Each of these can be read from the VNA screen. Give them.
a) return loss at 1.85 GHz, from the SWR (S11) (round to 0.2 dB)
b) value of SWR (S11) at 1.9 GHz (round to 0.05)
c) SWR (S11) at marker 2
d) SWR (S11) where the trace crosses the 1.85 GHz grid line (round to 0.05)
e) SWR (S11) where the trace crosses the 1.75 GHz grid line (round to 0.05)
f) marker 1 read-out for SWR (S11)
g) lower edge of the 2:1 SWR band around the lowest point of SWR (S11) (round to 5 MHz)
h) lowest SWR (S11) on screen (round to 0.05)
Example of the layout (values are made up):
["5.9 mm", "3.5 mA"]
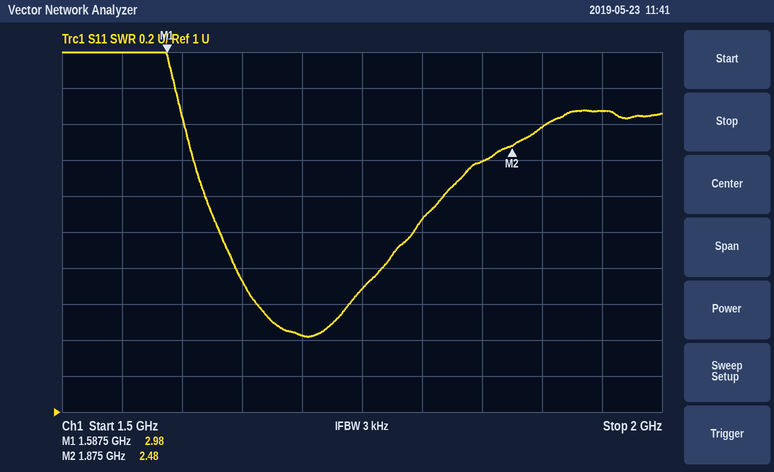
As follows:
["7.8 dB", "2.60", "2.48", "2.40", "1.70", "2.98", "1.630 GHz", "1.40"]
